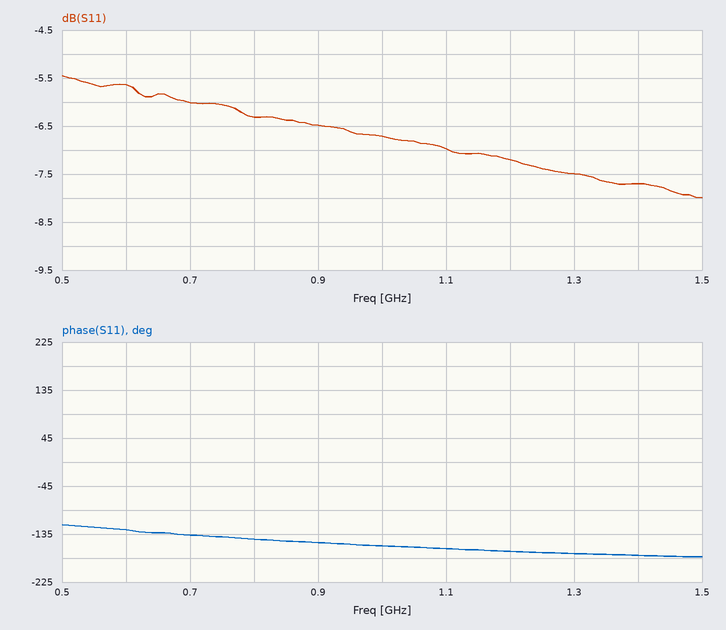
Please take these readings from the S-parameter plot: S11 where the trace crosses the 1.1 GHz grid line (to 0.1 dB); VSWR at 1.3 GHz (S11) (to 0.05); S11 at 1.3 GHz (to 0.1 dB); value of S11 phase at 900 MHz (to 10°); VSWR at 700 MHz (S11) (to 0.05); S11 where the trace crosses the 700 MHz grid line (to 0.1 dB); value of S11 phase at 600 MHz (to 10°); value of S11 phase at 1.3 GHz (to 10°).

-7.0 dB
2.45
-7.5 dB
-150°
3.00
-6.0 dB
-130°
-170°
